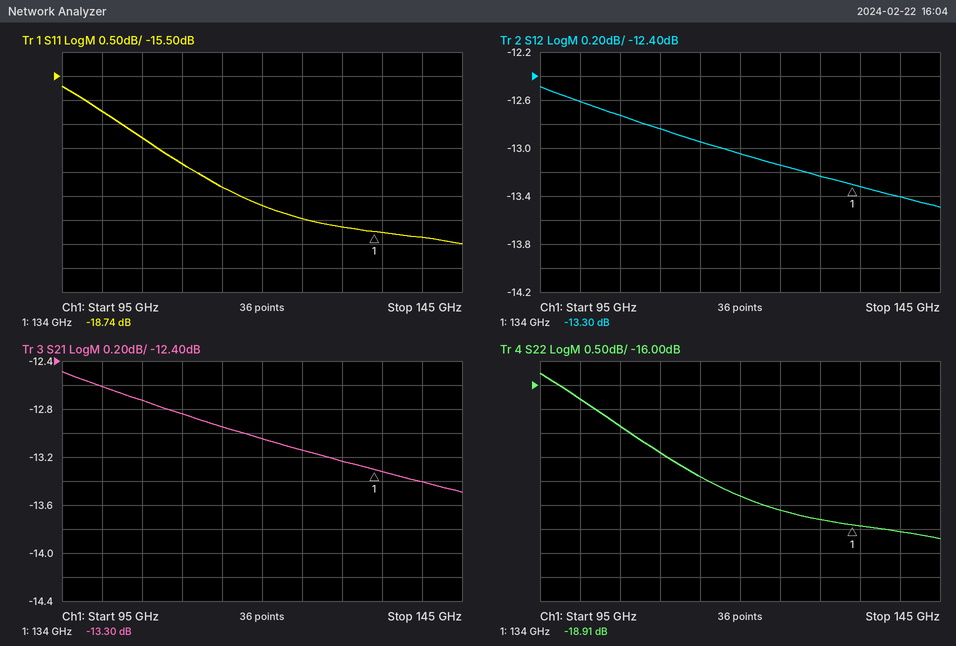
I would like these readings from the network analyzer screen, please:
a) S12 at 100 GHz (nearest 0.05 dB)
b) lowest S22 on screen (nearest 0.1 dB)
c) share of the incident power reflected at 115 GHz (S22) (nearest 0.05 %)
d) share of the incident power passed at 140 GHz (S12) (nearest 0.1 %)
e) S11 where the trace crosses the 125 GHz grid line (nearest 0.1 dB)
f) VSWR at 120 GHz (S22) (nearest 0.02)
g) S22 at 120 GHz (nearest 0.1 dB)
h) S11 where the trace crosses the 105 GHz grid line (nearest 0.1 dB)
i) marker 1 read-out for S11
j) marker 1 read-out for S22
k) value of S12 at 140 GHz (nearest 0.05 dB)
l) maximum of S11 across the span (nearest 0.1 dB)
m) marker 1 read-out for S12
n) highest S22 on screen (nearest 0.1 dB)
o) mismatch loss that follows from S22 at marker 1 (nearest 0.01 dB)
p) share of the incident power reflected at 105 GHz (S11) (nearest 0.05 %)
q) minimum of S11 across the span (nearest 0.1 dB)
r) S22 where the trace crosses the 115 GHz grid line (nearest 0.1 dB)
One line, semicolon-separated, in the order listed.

-12.60 dB; -19.2 dB; 1.60 %; 4.6 %; -18.5 dB; 1.28; -18.3 dB; -16.8 dB; -18.74 dB; -18.91 dB; -13.40 dB; -15.7 dB; -13.30 dB; -15.8 dB; 0.06 dB; 2.10 %; -19.0 dB; -17.9 dB
